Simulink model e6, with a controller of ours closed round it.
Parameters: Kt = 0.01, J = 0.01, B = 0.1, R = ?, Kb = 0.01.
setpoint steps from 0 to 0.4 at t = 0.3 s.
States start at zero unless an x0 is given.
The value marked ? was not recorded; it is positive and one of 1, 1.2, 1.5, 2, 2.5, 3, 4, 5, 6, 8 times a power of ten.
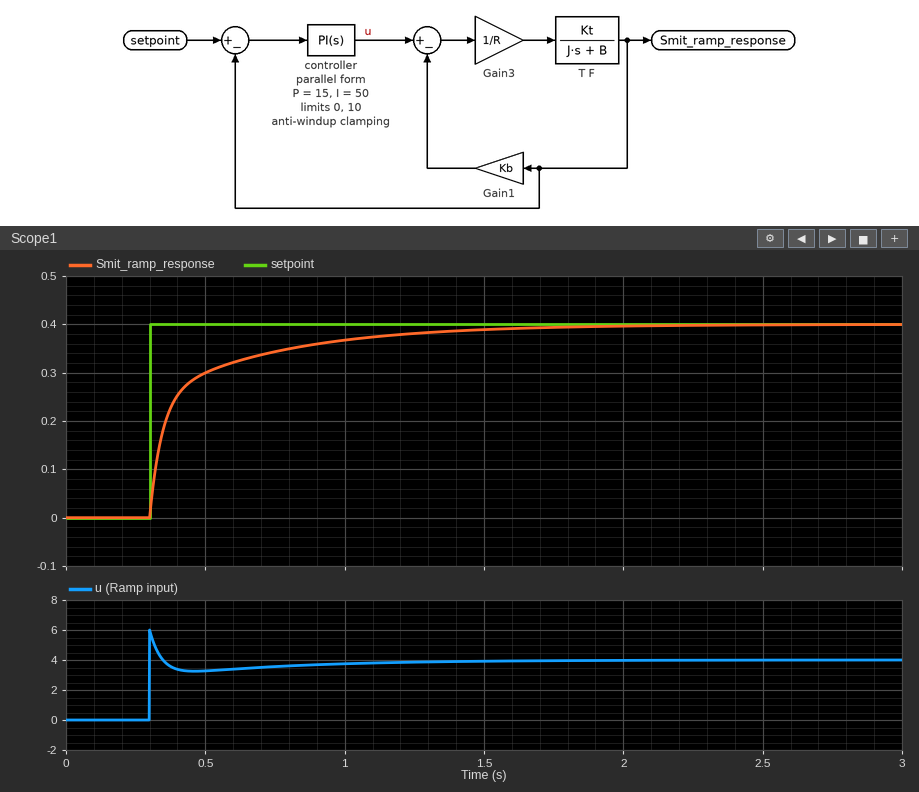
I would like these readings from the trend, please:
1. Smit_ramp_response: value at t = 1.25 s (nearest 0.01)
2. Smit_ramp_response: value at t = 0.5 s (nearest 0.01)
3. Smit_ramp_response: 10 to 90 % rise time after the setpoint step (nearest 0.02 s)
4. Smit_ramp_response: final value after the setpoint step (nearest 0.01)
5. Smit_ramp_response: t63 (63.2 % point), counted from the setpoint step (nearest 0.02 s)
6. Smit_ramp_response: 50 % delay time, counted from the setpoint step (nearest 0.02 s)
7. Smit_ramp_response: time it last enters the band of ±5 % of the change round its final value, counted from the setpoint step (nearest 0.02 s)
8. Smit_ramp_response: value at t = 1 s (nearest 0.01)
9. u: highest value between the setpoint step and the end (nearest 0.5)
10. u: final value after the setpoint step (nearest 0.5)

0.38
0.30
0.60 s
0.40
0.10 s
0.06 s
0.92 s
0.37
6.0
4.0
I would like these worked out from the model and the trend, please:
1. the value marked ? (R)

1
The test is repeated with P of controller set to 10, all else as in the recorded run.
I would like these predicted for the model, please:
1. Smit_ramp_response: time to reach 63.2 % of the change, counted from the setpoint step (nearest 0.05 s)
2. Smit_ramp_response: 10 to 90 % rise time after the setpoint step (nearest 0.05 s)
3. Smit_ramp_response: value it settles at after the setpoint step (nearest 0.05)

0.15 s
0.55 s
0.40
